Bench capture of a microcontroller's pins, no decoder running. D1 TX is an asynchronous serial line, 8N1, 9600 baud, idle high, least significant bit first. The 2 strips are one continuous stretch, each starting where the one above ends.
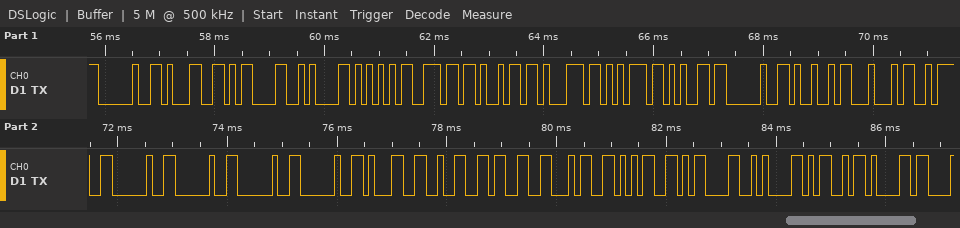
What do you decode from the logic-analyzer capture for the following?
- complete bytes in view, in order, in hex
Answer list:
20 31 0D 0A 55 6E 69 71 75 65 20 49 44 3A 20 20 20 20 31 32 33 34 35 0D 0A 4D 61
